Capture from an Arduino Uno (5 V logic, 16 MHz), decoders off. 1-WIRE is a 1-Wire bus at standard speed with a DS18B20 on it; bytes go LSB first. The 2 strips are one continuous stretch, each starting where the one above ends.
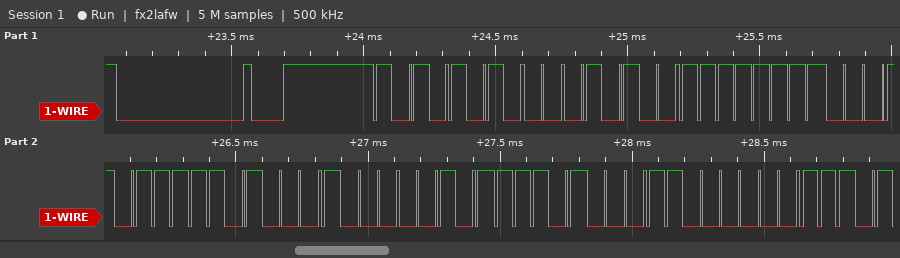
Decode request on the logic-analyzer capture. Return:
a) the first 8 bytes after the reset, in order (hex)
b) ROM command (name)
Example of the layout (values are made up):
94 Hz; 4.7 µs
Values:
55 28 FF E8 8B A0 17 03; Match ROM
